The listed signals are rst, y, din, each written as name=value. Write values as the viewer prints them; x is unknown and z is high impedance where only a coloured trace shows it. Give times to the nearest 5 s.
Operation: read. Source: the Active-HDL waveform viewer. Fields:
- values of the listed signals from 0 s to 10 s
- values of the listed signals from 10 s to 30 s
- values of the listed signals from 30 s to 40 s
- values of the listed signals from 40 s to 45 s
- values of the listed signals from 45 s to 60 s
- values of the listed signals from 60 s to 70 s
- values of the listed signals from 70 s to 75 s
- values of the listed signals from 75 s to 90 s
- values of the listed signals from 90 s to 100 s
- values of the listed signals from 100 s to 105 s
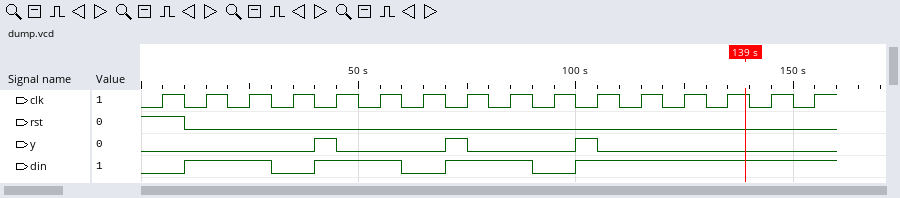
rst=1, y=0, din=0
rst=0, y=0, din=1
rst=0, y=0, din=0
rst=0, y=1, din=1
rst=0, y=0, din=1
rst=0, y=0, din=0
rst=0, y=1, din=1
rst=0, y=0, din=1
rst=0, y=0, din=0
rst=0, y=1, din=1
